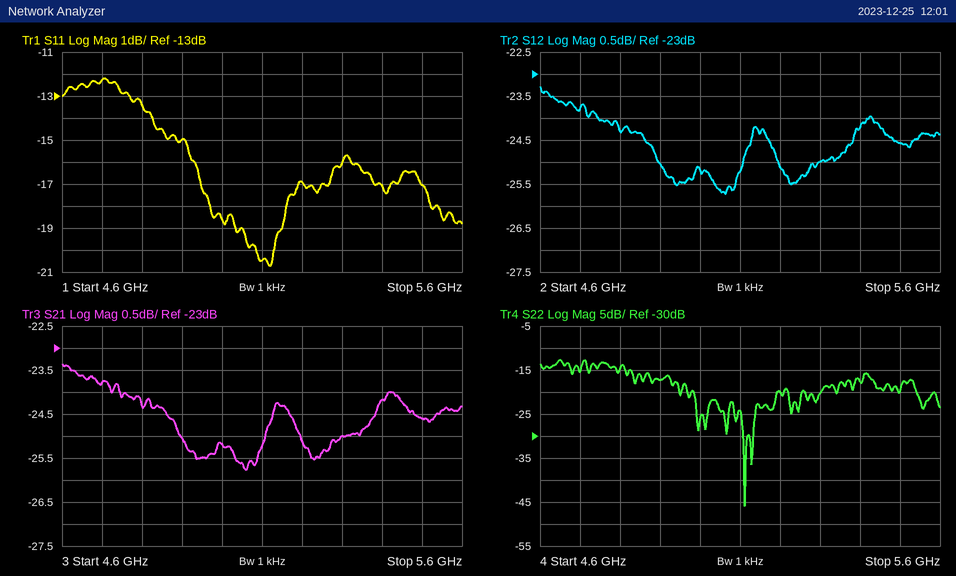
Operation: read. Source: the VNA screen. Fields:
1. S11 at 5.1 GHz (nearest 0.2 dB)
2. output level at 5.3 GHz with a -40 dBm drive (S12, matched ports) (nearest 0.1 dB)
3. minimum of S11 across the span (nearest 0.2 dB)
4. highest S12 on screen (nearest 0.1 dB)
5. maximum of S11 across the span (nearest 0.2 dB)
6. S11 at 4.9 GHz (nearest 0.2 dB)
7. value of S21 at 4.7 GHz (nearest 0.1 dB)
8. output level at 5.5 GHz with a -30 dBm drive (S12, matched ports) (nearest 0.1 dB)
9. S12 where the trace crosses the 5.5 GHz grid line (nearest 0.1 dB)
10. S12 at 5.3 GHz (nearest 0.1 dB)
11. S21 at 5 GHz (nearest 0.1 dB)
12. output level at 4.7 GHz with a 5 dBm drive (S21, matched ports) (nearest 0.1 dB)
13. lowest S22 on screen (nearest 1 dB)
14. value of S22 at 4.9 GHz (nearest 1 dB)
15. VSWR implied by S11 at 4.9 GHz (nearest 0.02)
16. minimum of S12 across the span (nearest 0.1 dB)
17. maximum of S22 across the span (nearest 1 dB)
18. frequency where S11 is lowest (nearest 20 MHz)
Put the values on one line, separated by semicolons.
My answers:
-20.4 dB; -65.0 dBm; -20.8 dB; -23.3 dB; -12.2 dB; -15.0 dB; -23.8 dB; -54.6 dBm; -24.6 dB; -25.0 dB; -25.2 dB; -18.8 dBm; -46 dB; -17 dB; 1.44; -25.7 dB; -13 dB; 5.12 GHz
